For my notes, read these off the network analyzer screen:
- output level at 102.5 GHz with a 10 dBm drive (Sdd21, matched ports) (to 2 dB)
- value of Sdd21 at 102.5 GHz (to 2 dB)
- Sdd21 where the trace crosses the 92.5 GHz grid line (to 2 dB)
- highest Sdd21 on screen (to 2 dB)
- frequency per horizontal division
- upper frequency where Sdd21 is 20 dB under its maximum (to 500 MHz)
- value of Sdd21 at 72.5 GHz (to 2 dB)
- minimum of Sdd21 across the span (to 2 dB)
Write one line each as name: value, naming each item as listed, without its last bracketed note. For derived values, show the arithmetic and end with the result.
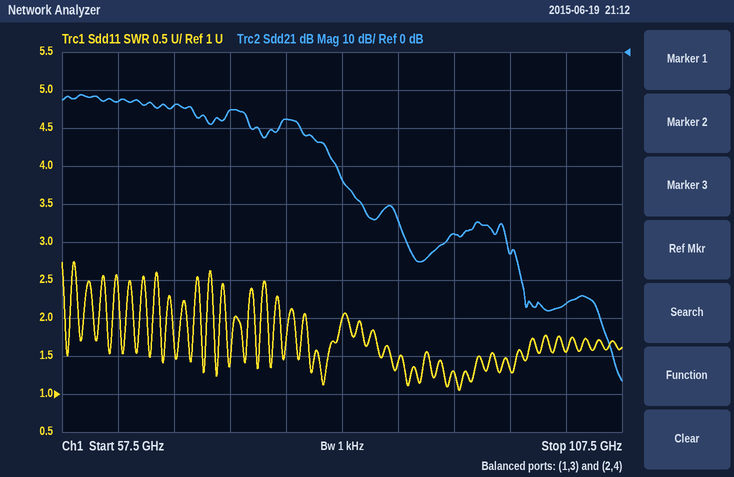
output level at 102.5 GHz with a 10 dBm drive (Sdd21, matched ports): 10 dBm + (-66 dB) = -56 dBm
value of Sdd21 at 102.5 GHz: -66 dB
Sdd21 where the trace crosses the 92.5 GHz grid line: -48 dB
highest Sdd21 on screen: -12 dB
frequency per horizontal division: 5 GHz
upper frequency where Sdd21 is 20 dB under its maximum: 82.0 GHz
value of Sdd21 at 72.5 GHz: -16 dB
minimum of Sdd21 across the span: -86 dB
